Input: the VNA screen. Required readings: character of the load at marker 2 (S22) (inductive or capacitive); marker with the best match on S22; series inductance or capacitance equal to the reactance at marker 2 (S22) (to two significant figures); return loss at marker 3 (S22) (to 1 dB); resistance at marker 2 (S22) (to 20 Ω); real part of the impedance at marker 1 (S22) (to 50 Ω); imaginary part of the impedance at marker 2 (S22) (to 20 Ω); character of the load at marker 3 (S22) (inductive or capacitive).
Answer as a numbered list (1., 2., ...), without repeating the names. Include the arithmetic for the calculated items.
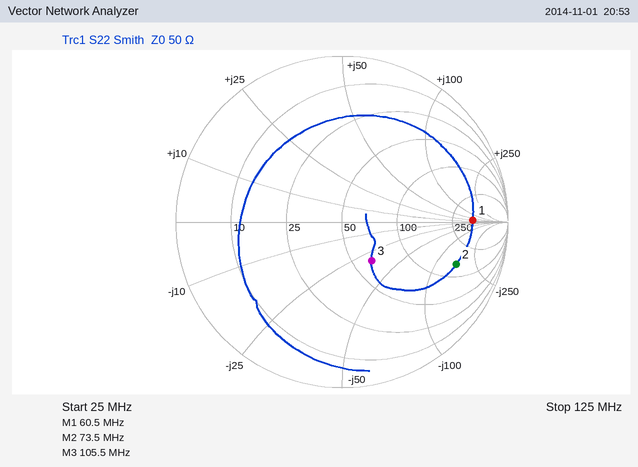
1. capacitive
2. marker 3
3. C = 1/(2π × 73.5 MHz × 160 Ω) ≈ 14 pF
4. 11 dB
5. 140 Ω
6. 400 Ω
7. -160 Ω
8. capacitive
